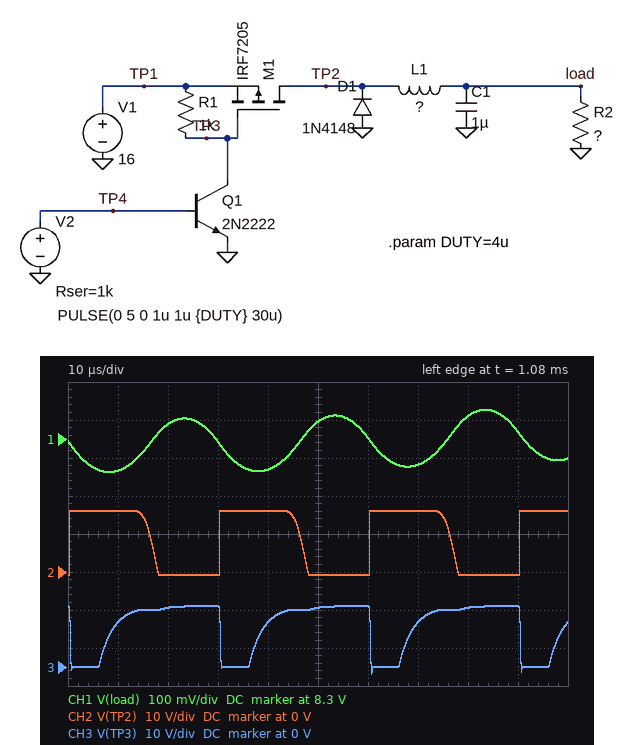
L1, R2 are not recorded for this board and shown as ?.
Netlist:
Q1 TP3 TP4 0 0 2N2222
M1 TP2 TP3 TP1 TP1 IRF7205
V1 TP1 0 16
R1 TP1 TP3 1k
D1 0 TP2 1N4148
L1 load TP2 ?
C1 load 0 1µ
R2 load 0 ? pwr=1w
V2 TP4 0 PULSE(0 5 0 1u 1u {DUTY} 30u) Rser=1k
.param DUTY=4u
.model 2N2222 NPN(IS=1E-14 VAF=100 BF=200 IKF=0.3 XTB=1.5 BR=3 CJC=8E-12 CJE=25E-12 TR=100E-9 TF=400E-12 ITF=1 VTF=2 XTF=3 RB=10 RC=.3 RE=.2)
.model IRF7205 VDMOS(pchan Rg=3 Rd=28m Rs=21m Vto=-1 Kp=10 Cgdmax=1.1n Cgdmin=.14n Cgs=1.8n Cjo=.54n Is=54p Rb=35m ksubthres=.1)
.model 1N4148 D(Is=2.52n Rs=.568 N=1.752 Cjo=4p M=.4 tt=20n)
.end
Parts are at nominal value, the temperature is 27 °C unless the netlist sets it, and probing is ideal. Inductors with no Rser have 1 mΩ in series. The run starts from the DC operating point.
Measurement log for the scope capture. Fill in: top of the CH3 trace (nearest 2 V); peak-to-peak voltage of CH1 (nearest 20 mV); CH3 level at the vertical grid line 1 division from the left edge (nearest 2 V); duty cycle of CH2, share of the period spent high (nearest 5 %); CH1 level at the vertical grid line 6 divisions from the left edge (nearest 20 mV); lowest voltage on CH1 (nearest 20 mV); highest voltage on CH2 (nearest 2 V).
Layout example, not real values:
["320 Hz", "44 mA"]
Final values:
["16 V", "160 mV", "12 V", "55 %", "8.30 V", "8.22 V", "16 V"]
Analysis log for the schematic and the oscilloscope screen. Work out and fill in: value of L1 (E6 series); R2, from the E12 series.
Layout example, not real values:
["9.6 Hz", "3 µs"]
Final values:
["3.3 mH", "120 Ω"]
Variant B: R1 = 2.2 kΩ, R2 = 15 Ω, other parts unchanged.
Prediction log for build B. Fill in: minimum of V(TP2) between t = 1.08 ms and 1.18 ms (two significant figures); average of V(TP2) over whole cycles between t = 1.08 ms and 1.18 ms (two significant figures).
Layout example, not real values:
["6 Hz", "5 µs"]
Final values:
["-1.4 V", "14 V"]
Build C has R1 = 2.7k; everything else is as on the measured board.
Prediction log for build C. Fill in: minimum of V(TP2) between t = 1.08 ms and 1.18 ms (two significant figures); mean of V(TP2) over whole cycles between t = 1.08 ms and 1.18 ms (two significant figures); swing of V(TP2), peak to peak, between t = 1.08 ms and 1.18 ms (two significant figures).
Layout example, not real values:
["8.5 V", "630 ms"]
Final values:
["14 V", "16 V", "1.8 V"]
